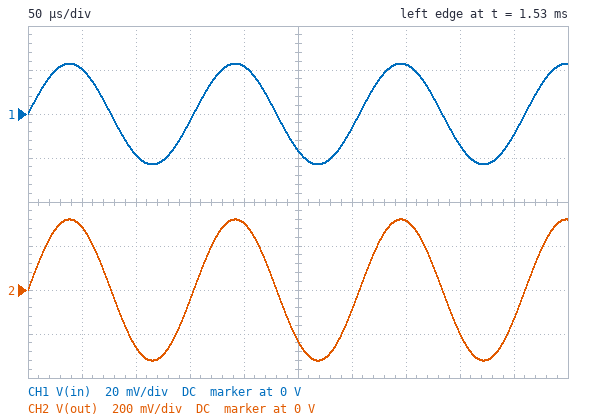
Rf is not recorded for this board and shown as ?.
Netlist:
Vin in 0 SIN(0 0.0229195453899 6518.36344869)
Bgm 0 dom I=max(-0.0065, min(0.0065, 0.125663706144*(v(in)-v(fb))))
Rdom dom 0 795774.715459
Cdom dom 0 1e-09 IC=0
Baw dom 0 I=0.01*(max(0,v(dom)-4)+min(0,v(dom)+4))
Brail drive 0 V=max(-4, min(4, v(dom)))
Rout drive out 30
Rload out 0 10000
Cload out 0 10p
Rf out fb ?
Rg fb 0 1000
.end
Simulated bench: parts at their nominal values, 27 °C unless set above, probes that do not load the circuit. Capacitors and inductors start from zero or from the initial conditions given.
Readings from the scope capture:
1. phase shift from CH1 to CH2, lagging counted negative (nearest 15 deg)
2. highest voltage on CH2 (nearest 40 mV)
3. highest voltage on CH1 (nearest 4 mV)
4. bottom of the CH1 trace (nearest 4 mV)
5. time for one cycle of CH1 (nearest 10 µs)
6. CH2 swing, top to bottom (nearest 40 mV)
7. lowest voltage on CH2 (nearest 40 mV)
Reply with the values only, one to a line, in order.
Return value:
0 deg
320 mV
24 mV
-24 mV
150 µs
640 mV
-320 mV
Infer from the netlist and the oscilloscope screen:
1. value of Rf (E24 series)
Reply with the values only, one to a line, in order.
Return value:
13 kΩ
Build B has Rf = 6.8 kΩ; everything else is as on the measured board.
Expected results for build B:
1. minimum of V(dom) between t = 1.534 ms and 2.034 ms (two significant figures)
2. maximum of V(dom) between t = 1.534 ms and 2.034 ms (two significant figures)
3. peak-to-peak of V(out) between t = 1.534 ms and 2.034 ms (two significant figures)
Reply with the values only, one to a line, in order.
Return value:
-180 mV
180 mV
360 mV
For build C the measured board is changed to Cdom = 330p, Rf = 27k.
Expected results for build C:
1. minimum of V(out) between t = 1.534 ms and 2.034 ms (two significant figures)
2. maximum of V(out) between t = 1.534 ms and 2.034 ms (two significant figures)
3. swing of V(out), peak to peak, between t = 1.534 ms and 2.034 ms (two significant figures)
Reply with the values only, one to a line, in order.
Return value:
-640 mV
640 mV
1.3 V
